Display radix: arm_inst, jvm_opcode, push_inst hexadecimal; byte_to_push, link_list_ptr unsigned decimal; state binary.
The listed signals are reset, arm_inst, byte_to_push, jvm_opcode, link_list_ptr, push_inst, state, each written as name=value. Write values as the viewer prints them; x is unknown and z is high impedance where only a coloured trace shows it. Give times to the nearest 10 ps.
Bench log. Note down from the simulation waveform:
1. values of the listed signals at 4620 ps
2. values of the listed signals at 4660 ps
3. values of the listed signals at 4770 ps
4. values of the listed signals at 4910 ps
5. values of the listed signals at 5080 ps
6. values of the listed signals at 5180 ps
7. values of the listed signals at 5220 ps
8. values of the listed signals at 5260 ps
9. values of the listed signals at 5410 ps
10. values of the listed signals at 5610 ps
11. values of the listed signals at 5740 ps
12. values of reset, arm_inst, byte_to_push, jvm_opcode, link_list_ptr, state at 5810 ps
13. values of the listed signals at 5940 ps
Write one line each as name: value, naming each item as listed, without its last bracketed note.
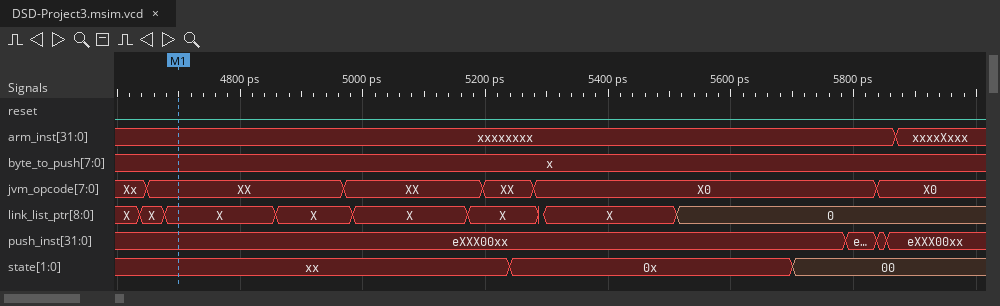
values of the listed signals at 4620 ps: reset=0, arm_inst=xxxxxxxx, byte_to_push=x, jvm_opcode=Xx, link_list_ptr=X, push_inst=eXXX00xx, state=xx
values of the listed signals at 4660 ps: reset=0, arm_inst=xxxxxxxx, byte_to_push=x, jvm_opcode=XX, link_list_ptr=X, push_inst=eXXX00xx, state=xx
values of the listed signals at 4770 ps: reset=0, arm_inst=xxxxxxxx, byte_to_push=x, jvm_opcode=XX, link_list_ptr=X, push_inst=eXXX00xx, state=xx
values of the listed signals at 4910 ps: reset=0, arm_inst=xxxxxxxx, byte_to_push=x, jvm_opcode=XX, link_list_ptr=X, push_inst=eXXX00xx, state=xx
values of the listed signals at 5080 ps: reset=0, arm_inst=xxxxxxxx, byte_to_push=x, jvm_opcode=XX, link_list_ptr=X, push_inst=eXXX00xx, state=xx
values of the listed signals at 5180 ps: reset=0, arm_inst=xxxxxxxx, byte_to_push=x, jvm_opcode=XX, link_list_ptr=X, push_inst=eXXX00xx, state=xx
values of the listed signals at 5220 ps: reset=0, arm_inst=xxxxxxxx, byte_to_push=x, jvm_opcode=XX, link_list_ptr=X, push_inst=eXXX00xx, state=xx
values of the listed signals at 5260 ps: reset=0, arm_inst=xxxxxxxx, byte_to_push=x, jvm_opcode=XX, link_list_ptr=X, push_inst=eXXX00xx, state=0x
values of the listed signals at 5410 ps: reset=0, arm_inst=xxxxxxxx, byte_to_push=x, jvm_opcode=X0, link_list_ptr=X, push_inst=eXXX00xx, state=0x
values of the listed signals at 5610 ps: reset=0, arm_inst=xxxxxxxx, byte_to_push=x, jvm_opcode=X0, link_list_ptr=0, push_inst=eXXX00xx, state=0x
values of the listed signals at 5740 ps: reset=0, arm_inst=xxxxxxxx, byte_to_push=x, jvm_opcode=X0, link_list_ptr=0, push_inst=eXXX00xx, state=00
values of reset, arm_inst, byte_to_push, jvm_opcode, link_list_ptr, state at 5810 ps: reset=0, arm_inst=xxxxxxxx, byte_to_push=x, jvm_opcode=X0, link_list_ptr=0, state=00
values of the listed signals at 5940 ps: reset=0, arm_inst=xxxxXxxx, byte_to_push=x, jvm_opcode=X0, link_list_ptr=0, push_inst=eXXX00xx, state=00
